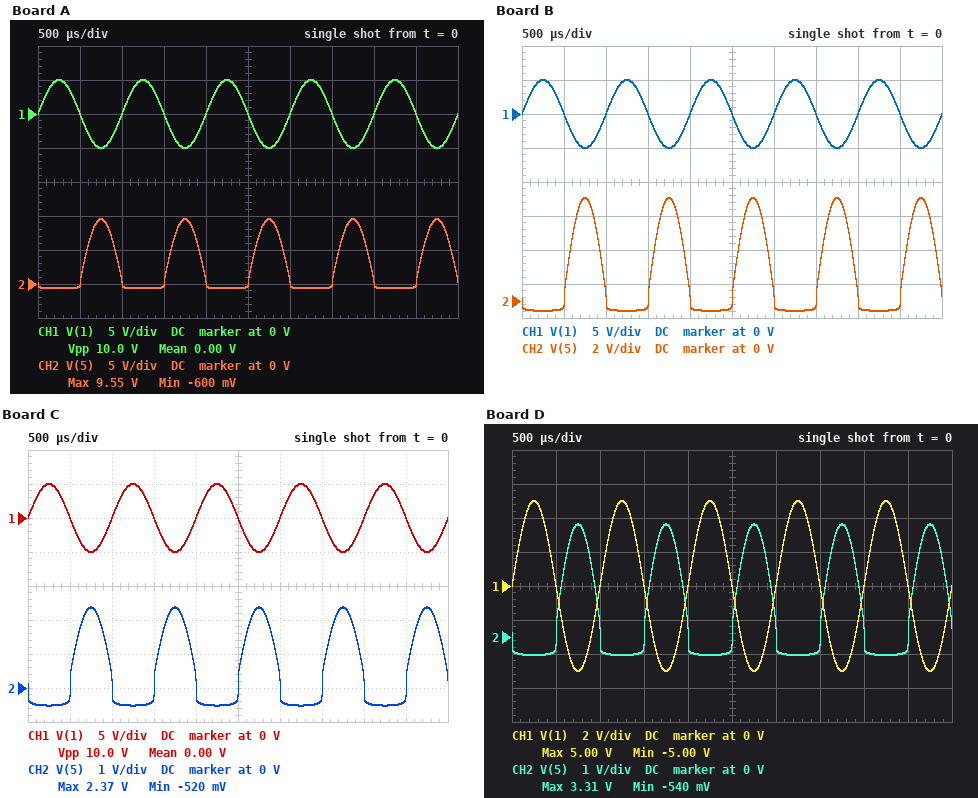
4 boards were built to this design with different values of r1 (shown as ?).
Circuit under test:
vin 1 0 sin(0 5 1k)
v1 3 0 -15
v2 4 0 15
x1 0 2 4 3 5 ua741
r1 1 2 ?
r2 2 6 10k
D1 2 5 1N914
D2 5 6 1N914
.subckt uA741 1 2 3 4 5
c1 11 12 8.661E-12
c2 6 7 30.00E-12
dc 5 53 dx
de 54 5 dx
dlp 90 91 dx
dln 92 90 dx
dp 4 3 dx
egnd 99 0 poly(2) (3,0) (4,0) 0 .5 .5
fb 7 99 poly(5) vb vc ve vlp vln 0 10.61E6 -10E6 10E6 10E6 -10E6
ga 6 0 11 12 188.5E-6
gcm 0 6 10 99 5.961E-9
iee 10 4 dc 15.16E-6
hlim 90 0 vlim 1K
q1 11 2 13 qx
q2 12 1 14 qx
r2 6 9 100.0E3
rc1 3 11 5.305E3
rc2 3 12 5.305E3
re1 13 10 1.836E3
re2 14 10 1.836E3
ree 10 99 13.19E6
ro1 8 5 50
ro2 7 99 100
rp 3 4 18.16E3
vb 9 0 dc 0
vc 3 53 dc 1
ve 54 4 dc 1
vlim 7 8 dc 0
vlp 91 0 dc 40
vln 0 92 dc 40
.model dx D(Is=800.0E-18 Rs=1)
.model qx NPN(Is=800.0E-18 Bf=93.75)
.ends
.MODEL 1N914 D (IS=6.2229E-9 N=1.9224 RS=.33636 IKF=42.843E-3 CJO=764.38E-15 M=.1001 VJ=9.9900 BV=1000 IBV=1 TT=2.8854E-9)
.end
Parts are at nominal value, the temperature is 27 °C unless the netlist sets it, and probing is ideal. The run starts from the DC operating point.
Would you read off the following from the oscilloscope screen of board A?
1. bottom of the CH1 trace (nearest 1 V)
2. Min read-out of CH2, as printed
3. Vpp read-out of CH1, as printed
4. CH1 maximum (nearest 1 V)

-5 V
-600 mV
10.0 V
5 V
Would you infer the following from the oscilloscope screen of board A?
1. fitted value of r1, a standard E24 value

5.6 kΩ
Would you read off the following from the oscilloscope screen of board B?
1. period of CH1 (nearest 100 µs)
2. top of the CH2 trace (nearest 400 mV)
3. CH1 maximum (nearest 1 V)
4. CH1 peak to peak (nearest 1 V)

1.0 ms
6.0 V
5 V
10 V
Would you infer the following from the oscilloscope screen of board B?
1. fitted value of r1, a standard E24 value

9.1 kΩ
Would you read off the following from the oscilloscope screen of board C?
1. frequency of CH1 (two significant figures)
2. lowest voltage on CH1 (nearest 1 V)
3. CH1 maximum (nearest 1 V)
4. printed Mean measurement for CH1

1.0 kHz
-5 V
5 V
0.00 V
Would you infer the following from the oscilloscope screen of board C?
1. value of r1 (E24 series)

27 kΩ
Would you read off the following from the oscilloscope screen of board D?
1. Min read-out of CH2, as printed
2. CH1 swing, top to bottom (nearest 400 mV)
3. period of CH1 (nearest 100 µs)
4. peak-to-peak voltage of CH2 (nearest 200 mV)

-540 mV
10.0 V
1.0 ms
3.8 V
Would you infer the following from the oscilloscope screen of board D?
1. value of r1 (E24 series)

18 kΩ
